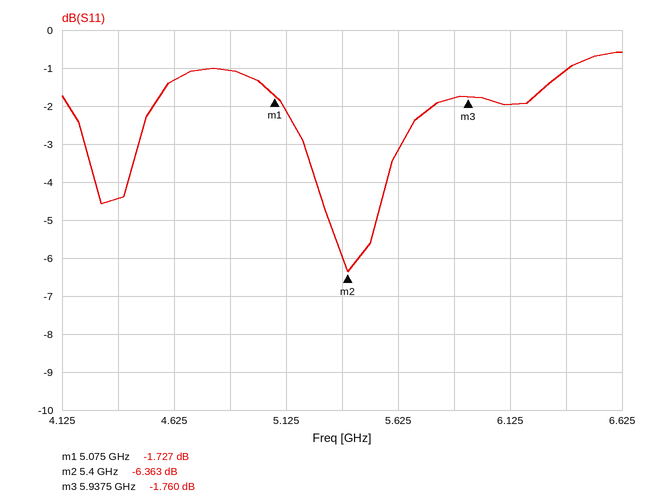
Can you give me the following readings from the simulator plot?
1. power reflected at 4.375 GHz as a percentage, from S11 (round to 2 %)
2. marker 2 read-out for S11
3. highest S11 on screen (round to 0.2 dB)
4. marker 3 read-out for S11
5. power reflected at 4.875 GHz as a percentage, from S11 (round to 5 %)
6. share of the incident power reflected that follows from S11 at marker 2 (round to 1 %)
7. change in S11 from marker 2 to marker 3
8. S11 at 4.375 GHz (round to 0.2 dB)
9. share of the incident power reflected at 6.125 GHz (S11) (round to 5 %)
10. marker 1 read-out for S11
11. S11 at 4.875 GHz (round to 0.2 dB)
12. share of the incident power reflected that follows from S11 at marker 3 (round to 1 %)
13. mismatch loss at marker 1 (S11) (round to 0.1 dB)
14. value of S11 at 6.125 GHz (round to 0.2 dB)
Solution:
36 %
-6.363 dB
-0.6 dB
-1.760 dB
80 %
23 %
4.603 dB
-4.4 dB
65 %
-1.727 dB
-1.0 dB
67 %
4.8 dB
-2.0 dB
